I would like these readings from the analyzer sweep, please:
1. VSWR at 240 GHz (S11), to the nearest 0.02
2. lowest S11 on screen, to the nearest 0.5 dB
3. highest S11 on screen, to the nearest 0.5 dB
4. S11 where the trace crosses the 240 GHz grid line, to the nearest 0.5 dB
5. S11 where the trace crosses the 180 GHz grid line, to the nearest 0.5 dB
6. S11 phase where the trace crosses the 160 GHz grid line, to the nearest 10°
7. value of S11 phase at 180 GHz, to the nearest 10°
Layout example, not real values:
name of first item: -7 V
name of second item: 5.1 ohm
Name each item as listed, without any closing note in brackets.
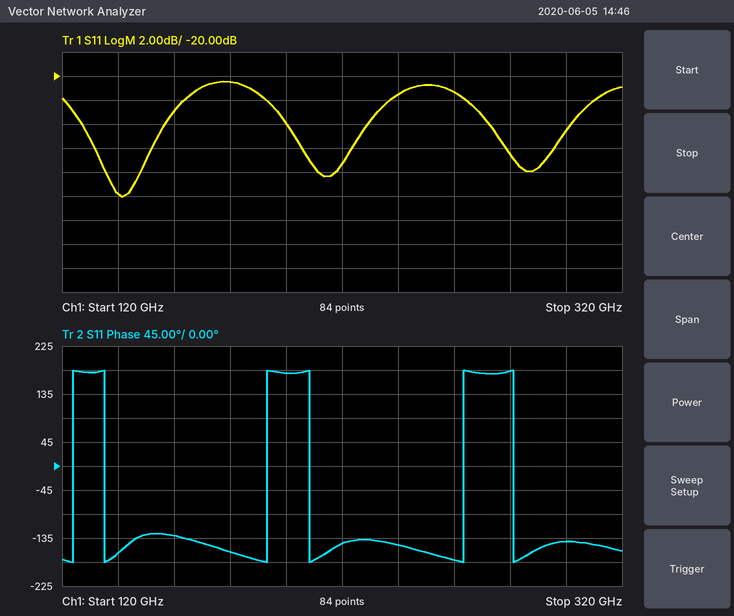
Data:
VSWR at 240 GHz (S11), to the nearest 0.02: 1.18
lowest S11 on screen, to the nearest 0.5 dB: -30.0 dB
highest S11 on screen, to the nearest 0.5 dB: -20.5 dB
S11 where the trace crosses the 240 GHz grid line, to the nearest 0.5 dB: -21.5 dB
S11 where the trace crosses the 180 GHz grid line, to the nearest 0.5 dB: -20.5 dB
S11 phase where the trace crosses the 160 GHz grid line, to the nearest 10°: -130°
value of S11 phase at 180 GHz, to the nearest 10°: -160°
